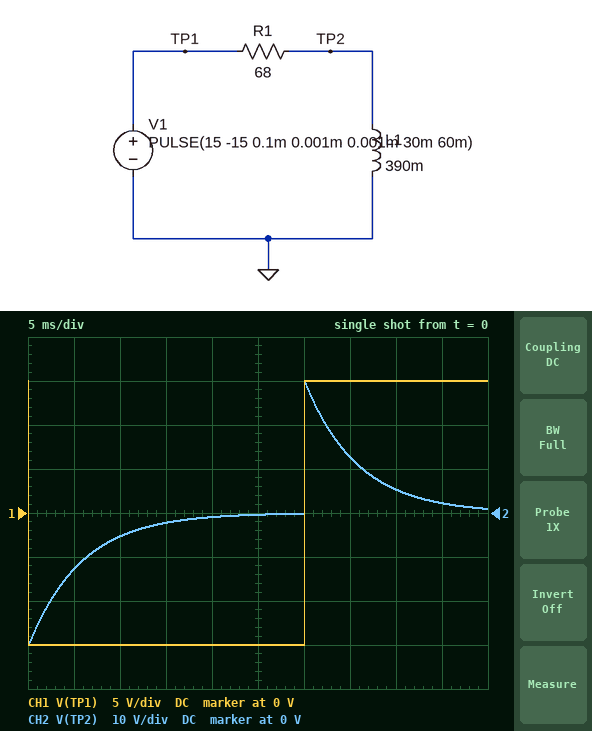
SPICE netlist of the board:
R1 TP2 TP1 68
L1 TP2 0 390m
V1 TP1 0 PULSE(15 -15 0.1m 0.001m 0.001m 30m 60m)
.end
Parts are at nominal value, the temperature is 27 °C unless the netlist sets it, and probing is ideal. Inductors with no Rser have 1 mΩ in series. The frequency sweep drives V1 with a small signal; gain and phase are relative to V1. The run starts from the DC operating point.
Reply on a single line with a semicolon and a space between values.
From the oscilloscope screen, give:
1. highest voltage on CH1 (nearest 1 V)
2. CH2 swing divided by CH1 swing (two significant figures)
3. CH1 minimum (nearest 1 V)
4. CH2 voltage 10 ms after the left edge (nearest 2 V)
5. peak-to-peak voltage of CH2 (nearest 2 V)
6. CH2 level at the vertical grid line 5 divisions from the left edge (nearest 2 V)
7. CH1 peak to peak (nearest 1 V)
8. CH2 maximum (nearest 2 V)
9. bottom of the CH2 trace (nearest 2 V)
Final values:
15 V; 2.0; -15 V; -6 V; 60 V; 0 V; 30 V; 30 V; -30 V
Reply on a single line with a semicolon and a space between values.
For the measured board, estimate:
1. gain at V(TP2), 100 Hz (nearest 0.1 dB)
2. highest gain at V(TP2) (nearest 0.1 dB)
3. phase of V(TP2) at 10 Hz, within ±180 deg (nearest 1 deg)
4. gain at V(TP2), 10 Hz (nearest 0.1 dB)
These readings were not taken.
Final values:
-0.3 dB; 0 dB; 70 deg; -9.4 dB
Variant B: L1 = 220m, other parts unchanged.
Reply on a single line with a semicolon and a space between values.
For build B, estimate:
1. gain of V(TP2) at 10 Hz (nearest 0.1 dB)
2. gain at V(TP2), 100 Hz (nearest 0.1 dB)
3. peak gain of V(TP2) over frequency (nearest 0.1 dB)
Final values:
-14.0 dB; -0.9 dB; 0 dB
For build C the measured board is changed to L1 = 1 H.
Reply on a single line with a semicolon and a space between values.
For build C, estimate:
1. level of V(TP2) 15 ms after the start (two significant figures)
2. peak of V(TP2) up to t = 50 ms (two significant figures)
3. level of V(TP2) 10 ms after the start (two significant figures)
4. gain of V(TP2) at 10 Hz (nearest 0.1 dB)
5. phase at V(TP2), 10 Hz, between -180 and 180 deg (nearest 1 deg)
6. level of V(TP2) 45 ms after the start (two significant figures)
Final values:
-11 V; 26 V; -15 V; -3.4 dB; 47 deg; 9.5 V
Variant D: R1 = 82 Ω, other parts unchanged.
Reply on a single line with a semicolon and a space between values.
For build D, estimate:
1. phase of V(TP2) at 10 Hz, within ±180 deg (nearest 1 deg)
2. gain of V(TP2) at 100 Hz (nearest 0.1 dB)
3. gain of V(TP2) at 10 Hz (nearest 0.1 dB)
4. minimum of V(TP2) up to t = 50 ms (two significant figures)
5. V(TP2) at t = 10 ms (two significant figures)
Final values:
73 deg; -0.5 dB; -10.9 dB; -30 V; -3.7 V
